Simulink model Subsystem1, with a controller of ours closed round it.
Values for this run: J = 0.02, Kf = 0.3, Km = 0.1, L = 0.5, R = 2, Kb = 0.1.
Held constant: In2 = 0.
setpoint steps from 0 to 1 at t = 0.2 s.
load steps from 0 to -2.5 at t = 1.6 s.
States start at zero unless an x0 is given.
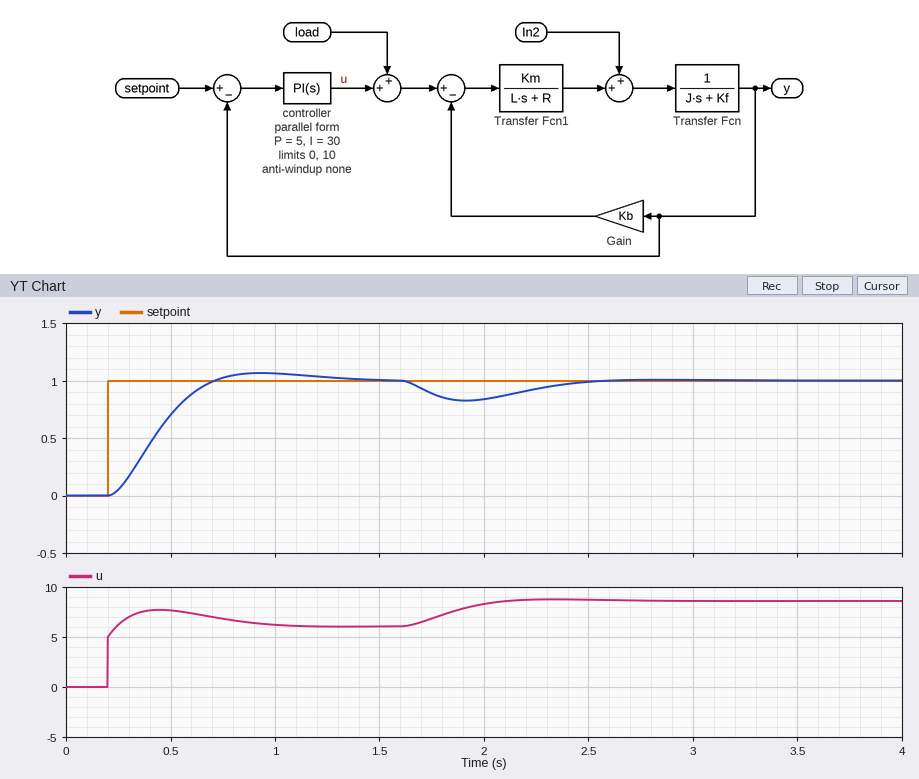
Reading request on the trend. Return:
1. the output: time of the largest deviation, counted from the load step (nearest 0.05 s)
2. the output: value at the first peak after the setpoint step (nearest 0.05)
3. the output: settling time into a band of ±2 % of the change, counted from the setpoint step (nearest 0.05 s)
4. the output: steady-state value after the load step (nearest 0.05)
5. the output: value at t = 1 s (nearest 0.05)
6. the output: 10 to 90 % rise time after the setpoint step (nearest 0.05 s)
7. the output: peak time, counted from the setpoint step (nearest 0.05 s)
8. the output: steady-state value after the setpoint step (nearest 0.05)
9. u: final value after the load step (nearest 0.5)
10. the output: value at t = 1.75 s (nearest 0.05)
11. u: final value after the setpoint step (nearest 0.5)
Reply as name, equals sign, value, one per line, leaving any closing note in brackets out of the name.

the output: time of the largest deviation, counted from the load step = 0.30 s
the output: value at the first peak after the setpoint step = 1.05
the output: settling time into a band of ±2 % of the change, counted from the setpoint step = 1.10 s
the output: steady-state value after the load step = 1.00
the output: value at t = 1 s = 1.05
the output: 10 to 90 % rise time after the setpoint step = 0.35 s
the output: peak time, counted from the setpoint step = 0.75 s
the output: steady-state value after the setpoint step = 1.00
u: final value after the load step = 8.5
the output: value at t = 1.75 s = 0.90
u: final value after the setpoint step = 6.0
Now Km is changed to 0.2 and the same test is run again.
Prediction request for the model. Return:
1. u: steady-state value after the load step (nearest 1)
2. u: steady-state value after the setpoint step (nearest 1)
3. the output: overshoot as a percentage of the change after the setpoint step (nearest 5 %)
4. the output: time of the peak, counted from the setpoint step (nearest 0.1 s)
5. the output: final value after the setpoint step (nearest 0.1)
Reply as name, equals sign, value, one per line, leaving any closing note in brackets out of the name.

u: steady-state value after the load step = 6
u: steady-state value after the setpoint step = 3
the output: overshoot as a percentage of the change after the setpoint step = 15 %
the output: time of the peak, counted from the setpoint step = 0.4 s
the output: final value after the setpoint step = 1.0
